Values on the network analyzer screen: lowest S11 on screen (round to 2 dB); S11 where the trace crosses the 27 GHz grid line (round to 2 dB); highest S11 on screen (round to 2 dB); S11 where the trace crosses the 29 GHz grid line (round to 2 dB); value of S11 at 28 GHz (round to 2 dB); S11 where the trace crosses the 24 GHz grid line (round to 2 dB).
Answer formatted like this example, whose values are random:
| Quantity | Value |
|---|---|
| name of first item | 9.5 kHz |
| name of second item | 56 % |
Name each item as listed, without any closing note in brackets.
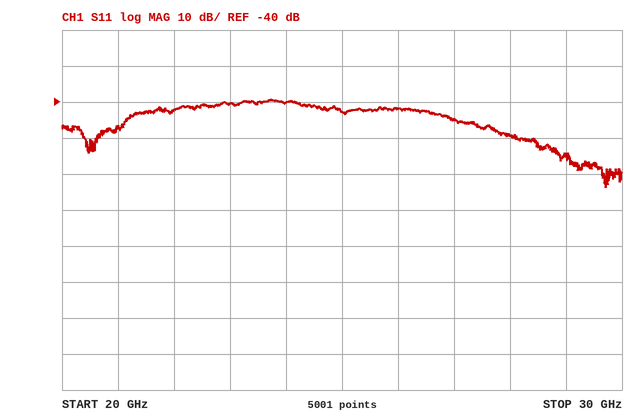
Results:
| Quantity | Value |
|---|---|
| lowest S11 on screen | -64 dB |
| S11 where the trace crosses the 27 GHz grid line | -44 dB |
| highest S11 on screen | -40 dB |
| S11 where the trace crosses the 29 GHz grid line | -54 dB |
| value of S11 at 28 GHz | -50 dB |
| S11 where the trace crosses the 24 GHz grid line | -40 dB |
